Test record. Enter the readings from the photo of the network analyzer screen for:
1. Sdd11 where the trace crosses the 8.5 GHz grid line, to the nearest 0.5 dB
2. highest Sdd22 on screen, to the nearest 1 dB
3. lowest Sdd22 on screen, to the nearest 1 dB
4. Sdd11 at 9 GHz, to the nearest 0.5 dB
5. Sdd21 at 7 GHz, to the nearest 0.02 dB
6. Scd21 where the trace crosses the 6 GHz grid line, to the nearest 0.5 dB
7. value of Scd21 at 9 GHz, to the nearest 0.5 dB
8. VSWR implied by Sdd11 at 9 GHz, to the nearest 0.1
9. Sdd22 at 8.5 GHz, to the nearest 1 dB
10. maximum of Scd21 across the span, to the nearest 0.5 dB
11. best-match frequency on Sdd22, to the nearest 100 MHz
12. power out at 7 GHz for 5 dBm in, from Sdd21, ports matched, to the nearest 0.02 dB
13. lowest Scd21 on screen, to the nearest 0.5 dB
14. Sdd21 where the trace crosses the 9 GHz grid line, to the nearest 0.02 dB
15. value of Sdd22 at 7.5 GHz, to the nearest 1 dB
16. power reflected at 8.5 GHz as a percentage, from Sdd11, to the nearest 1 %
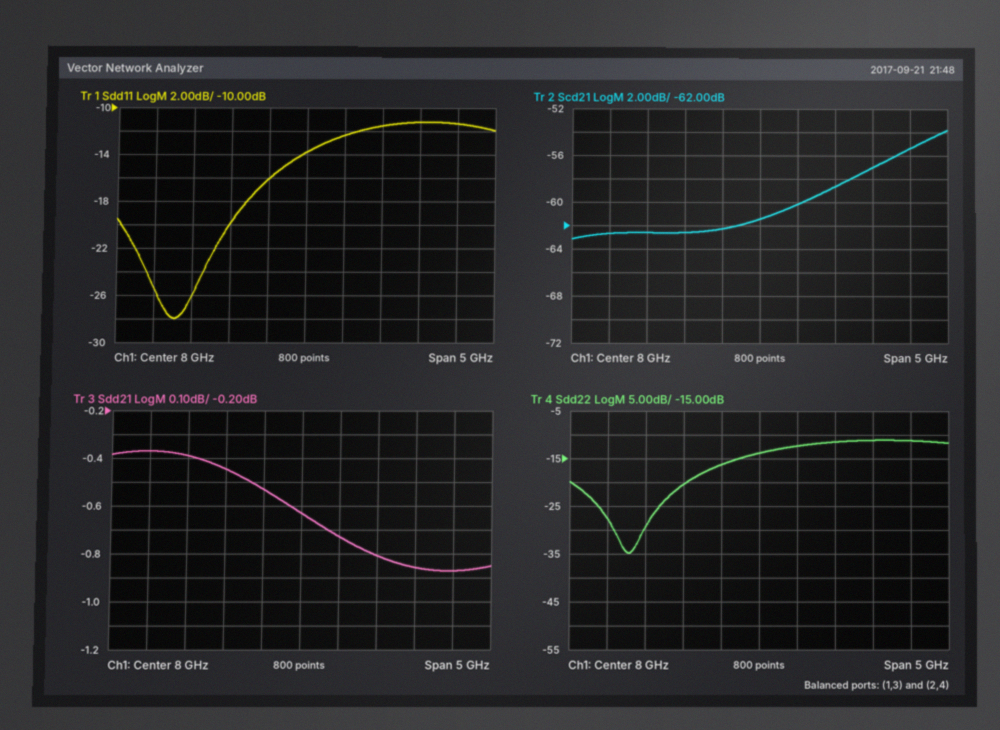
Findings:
-12.5 dB
-11 dB
-35 dB
-11.5 dB
-0.44 dB
-62.5 dB
-58.5 dB
1.7
-12 dB
-54.0 dB
6.3 GHz
4.56 dBm
-63.0 dB
-0.80 dB
-16 dB
6 %
